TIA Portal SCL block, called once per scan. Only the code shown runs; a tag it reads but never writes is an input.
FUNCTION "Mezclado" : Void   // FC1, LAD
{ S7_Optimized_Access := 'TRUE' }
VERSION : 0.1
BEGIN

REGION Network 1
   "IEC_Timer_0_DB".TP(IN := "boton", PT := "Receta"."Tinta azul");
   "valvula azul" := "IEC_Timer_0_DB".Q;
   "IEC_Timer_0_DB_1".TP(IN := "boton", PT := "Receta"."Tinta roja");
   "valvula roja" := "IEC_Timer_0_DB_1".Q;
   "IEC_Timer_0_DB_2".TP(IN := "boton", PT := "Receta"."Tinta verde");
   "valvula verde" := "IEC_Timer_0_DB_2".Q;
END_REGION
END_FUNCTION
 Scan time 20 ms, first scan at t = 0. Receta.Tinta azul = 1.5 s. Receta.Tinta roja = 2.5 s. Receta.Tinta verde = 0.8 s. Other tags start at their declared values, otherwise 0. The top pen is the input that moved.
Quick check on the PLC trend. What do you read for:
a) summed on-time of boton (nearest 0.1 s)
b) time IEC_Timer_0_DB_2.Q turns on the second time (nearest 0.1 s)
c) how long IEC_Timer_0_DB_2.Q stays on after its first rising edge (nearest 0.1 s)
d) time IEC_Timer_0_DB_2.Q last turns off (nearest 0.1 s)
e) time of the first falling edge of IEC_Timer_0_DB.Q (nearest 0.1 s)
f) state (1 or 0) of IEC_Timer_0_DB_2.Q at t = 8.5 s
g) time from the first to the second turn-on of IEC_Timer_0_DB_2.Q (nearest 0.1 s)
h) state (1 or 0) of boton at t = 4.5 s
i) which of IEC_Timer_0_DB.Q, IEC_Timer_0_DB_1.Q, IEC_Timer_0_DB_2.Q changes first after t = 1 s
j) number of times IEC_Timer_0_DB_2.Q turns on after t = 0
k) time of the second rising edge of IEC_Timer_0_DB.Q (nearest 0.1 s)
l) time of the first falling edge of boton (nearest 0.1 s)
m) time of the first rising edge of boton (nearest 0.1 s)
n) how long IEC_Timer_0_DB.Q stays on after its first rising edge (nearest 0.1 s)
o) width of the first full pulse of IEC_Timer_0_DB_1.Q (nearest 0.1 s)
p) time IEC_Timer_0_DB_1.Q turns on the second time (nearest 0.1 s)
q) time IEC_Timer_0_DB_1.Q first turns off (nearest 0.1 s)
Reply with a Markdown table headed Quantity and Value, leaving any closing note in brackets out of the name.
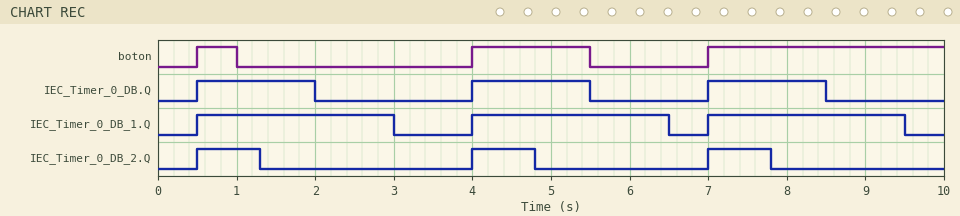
| Quantity | Value |
|---|---|
| summed on-time of boton | 5.0 s |
| time IEC_Timer_0_DB_2.Q turns on the second time | 4.0 s |
| how long IEC_Timer_0_DB_2.Q stays on after its first rising edge | 0.8 s |
| time IEC_Timer_0_DB_2.Q last turns off | 7.8 s |
| time of the first falling edge of IEC_Timer_0_DB.Q | 2.0 s |
| state (1 or 0) of IEC_Timer_0_DB_2.Q at t = 8.5 s | 0 |
| time from the first to the second turn-on of IEC_Timer_0_DB_2.Q | 3.5 s |
| state (1 or 0) of boton at t = 4.5 s | 1 |
| which of IEC_Timer_0_DB.Q, IEC_Timer_0_DB_1.Q, IEC_Timer_0_DB_2.Q changes first after t = 1 s | IEC_Timer_0_DB_2.Q |
| number of times IEC_Timer_0_DB_2.Q turns on after t = 0 | 3 |
| time of the second rising edge of IEC_Timer_0_DB.Q | 4.0 s |
| time of the first falling edge of boton | 1.0 s |
| time of the first rising edge of boton | 0.5 s |
| how long IEC_Timer_0_DB.Q stays on after its first rising edge | 1.5 s |
| width of the first full pulse of IEC_Timer_0_DB_1.Q | 2.5 s |
| time IEC_Timer_0_DB_1.Q turns on the second time | 4.0 s |
| time IEC_Timer_0_DB_1.Q first turns off | 3.0 s |
